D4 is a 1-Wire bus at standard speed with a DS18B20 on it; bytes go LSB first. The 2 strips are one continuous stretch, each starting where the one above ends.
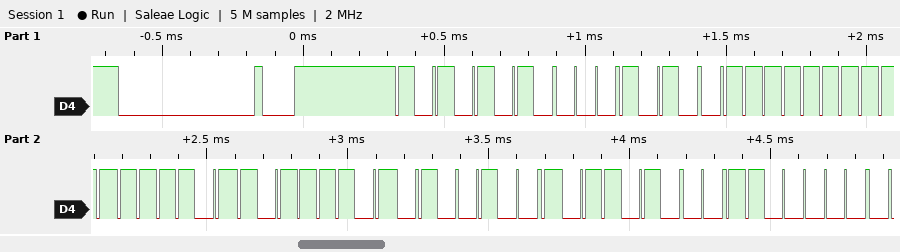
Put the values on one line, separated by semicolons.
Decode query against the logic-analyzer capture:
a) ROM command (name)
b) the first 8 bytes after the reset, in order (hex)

Match ROM; 55 28 FF BF BD 92 16 03
